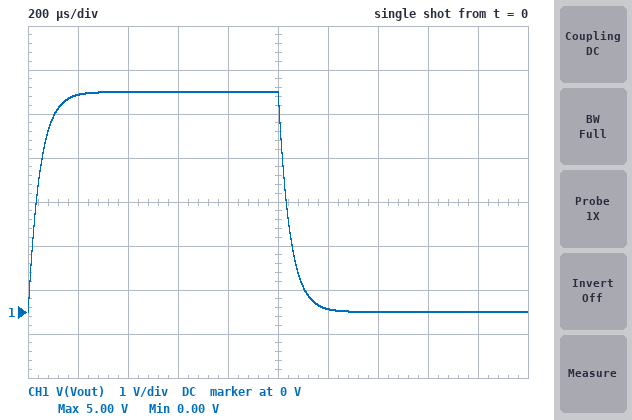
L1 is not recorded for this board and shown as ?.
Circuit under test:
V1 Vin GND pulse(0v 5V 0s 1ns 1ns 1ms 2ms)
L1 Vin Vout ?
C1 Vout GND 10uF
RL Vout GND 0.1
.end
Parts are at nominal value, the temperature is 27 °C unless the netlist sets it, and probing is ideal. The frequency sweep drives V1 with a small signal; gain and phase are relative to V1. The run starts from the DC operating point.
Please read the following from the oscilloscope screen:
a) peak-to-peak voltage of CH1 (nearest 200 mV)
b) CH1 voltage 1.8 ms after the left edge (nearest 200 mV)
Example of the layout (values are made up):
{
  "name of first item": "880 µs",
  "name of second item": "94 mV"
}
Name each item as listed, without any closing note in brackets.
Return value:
{
  "peak-to-peak voltage of CH1": "5.0 V",
  "CH1 voltage 1.8 ms after the left edge": "0 V"
}
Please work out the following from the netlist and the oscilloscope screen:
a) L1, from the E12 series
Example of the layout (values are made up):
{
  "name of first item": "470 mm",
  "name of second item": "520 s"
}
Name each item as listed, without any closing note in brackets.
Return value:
{
  "L1, from the E12 series": "4.7 µH"
}
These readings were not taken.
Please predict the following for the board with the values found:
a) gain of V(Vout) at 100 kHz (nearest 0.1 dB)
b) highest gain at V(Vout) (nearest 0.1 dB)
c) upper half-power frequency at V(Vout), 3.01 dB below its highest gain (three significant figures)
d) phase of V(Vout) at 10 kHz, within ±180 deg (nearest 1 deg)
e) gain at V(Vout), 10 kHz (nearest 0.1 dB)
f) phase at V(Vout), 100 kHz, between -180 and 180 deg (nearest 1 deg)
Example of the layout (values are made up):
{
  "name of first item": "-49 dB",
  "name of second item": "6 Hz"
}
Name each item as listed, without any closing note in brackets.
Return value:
{
  "gain of V(Vout) at 100 kHz": "-30.7 dB",
  "highest gain at V(Vout)": "0 dB",
  "upper half-power frequency at V(Vout), 3.01 dB below its highest gain": "3.46 kHz",
  "phase of V(Vout) at 10 kHz, within ±180 deg": "-75 deg",
  "gain at V(Vout), 10 kHz": "-9.7 dB",
  "phase at V(Vout), 100 kHz, between -180 and 180 deg": "-121 deg"
}
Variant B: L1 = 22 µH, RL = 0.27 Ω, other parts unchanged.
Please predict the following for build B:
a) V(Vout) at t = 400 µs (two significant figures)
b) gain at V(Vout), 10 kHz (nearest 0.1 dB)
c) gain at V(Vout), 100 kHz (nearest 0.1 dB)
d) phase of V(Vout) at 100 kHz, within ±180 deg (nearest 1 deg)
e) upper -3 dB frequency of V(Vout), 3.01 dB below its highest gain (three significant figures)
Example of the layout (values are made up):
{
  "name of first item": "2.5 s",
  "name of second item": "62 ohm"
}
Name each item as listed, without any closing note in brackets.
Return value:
{
  "V(Vout) at t = 400 µs": "5.0 V",
  "gain at V(Vout), 10 kHz": "-14.2 dB",
  "gain at V(Vout), 100 kHz": "-40.0 dB",
  "phase of V(Vout) at 100 kHz, within ±180 deg": "-149 deg",
  "upper -3 dB frequency of V(Vout), 3.01 dB below its highest gain": "2.02 kHz"
}
